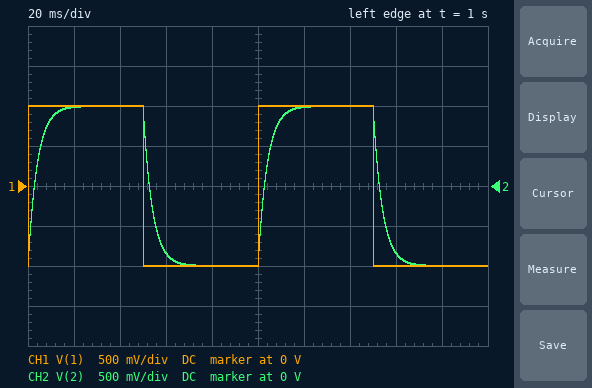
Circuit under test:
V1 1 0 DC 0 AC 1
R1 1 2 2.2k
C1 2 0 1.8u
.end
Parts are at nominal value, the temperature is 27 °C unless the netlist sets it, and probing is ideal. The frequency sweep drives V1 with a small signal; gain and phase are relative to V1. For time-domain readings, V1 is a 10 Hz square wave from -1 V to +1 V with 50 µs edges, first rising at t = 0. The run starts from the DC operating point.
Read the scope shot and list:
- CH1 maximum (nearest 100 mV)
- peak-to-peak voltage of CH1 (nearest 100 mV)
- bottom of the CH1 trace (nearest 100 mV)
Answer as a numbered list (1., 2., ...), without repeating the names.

1. 1.0 V
2. 2.0 V
3. -1.0 V
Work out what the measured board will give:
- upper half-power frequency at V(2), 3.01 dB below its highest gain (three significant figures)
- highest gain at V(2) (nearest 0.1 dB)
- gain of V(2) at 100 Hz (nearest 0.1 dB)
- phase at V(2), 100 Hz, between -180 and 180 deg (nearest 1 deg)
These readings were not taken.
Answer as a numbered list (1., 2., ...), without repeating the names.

1. 40.2 Hz
2. 0 dB
3. -8.6 dB
4. -68 deg
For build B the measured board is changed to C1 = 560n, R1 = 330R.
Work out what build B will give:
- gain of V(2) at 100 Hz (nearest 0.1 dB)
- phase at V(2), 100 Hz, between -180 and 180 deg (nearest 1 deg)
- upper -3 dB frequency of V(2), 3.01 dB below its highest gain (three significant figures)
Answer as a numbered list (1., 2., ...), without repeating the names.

1. -0.1 dB
2. -7 deg
3. 861 Hz
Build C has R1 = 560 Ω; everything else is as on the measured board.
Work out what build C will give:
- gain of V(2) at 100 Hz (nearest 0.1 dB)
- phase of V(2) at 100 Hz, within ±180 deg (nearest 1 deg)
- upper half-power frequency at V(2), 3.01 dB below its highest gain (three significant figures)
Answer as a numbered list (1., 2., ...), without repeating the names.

1. -1.5 dB
2. -32 deg
3. 158 Hz
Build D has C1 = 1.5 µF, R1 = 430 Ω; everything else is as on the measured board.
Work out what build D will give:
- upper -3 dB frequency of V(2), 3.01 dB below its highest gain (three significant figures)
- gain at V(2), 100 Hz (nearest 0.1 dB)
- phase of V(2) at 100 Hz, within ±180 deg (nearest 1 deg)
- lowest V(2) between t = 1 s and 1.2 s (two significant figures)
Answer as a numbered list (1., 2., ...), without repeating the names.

1. 247 Hz
2. -0.7 dB
3. -22 deg
4. -1.0 V
